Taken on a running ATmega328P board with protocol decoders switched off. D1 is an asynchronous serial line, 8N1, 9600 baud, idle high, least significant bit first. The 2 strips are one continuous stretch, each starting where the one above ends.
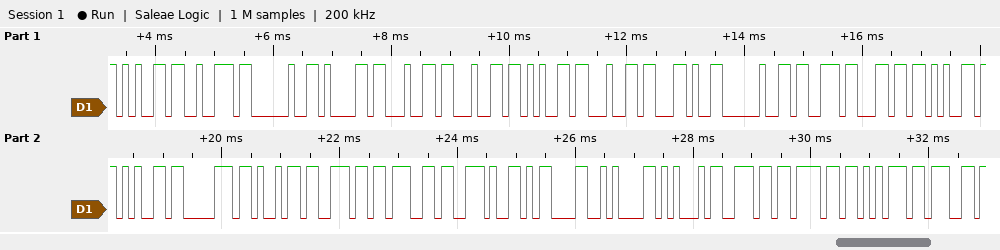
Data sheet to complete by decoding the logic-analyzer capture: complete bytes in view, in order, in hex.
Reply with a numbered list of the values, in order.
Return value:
1. 65 72 20 61 64 64 65 64 2C 20 73 6C 65 65 70 69 6E 67 2E 0D 0A 45 6E 6F 75 67
